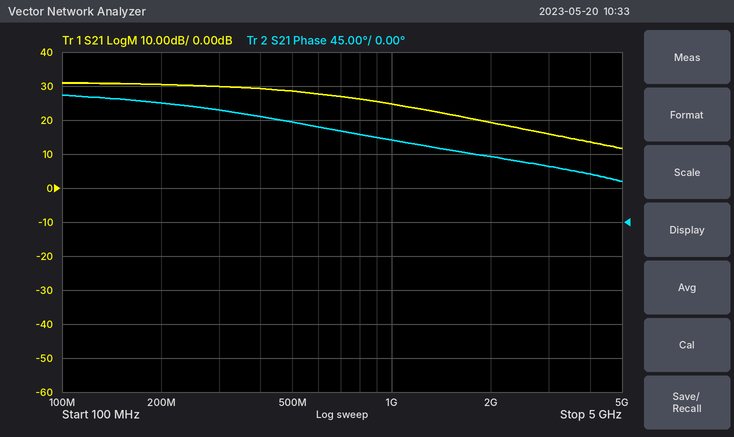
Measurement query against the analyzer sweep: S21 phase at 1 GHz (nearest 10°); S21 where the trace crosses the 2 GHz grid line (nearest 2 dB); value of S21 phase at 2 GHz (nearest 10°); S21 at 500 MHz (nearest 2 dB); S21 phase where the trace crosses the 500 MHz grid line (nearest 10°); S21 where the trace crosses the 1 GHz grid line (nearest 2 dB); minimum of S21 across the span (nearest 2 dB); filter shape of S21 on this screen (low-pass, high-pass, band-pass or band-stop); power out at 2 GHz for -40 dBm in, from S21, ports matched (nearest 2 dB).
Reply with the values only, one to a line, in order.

110°
20 dB
90°
28 dB
130°
24 dB
12 dB
low-pass
-20 dBm
